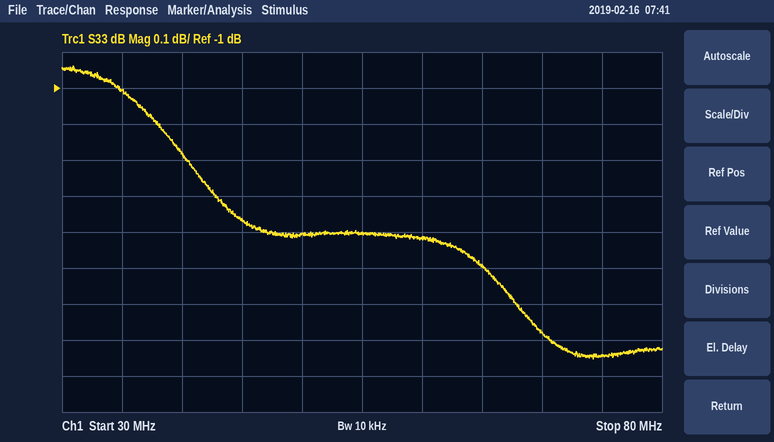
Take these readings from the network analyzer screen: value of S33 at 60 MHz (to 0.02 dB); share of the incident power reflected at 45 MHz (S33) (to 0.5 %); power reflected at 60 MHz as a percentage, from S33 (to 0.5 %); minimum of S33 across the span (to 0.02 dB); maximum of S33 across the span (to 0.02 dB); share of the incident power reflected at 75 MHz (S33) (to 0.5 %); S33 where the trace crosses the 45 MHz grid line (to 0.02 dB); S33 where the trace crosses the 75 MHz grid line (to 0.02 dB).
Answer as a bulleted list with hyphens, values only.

- -1.42 dB
- 73.0 %
- 72.0 %
- -1.76 dB
- -0.94 dB
- 67.0 %
- -1.36 dB
- -1.74 dB
